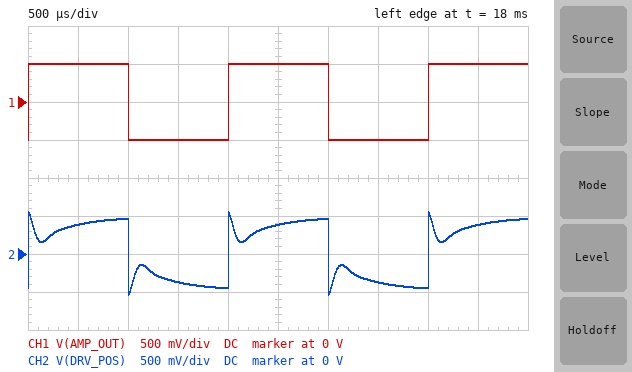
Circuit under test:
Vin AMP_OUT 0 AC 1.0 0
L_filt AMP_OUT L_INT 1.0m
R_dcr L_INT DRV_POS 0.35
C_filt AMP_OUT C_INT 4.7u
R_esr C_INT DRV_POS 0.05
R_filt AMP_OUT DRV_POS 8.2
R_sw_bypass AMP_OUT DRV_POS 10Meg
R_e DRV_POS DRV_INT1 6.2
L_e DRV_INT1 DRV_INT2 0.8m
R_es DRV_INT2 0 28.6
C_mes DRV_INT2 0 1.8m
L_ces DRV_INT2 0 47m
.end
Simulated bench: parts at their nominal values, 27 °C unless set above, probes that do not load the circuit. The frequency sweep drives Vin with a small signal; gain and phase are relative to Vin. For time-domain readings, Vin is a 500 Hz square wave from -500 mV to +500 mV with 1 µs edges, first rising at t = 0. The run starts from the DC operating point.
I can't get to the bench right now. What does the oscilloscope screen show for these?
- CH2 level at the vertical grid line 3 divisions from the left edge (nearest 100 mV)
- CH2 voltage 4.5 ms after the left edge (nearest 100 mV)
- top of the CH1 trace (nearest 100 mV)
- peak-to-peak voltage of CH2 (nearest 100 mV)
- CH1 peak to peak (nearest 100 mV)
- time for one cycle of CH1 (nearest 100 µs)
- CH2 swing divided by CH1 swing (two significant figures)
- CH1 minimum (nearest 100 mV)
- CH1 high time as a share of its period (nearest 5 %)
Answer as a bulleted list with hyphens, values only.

- -400 mV
- 400 mV
- 500 mV
- 1.1 V
- 1.0 V
- 2.0 ms
- 1.1
- -500 mV
- 50 %
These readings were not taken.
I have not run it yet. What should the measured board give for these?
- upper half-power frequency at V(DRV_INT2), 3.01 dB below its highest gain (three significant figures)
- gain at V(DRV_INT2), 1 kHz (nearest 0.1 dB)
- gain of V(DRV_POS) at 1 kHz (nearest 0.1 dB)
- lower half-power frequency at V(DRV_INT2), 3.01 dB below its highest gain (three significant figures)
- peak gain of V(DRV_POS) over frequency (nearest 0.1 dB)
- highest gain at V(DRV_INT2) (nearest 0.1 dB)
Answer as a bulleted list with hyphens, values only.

- 27.9 Hz
- -43.6 dB
- -4.5 dB
- 11.0 Hz
- 0.9 dB
- -1.8 dB
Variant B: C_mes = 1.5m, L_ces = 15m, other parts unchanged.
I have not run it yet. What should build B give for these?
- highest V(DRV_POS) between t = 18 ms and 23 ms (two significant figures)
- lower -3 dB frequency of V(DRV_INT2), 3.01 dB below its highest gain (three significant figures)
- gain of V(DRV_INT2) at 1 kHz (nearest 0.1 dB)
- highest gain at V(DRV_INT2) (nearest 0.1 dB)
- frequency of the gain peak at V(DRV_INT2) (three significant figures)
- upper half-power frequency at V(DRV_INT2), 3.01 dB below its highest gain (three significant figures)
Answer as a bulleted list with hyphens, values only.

- 540 mV
- 25.3 Hz
- -42.0 dB
- -1.8 dB
- 34.0 Hz
- 45.7 Hz
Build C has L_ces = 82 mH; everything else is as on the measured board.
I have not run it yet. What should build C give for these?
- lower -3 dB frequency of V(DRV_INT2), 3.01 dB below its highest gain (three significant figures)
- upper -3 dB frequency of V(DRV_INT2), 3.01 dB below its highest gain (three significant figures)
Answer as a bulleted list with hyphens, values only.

- 7.24 Hz
- 24.2 Hz
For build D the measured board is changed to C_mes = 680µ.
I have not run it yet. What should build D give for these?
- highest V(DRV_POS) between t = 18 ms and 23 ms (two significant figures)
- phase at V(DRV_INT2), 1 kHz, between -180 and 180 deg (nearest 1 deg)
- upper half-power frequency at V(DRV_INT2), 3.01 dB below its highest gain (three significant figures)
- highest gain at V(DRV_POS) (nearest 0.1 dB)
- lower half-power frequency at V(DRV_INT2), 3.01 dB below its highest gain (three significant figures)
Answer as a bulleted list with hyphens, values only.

- 540 mV
- -130 deg
- 60.4 Hz
- 0.9 dB
- 13.9 Hz
